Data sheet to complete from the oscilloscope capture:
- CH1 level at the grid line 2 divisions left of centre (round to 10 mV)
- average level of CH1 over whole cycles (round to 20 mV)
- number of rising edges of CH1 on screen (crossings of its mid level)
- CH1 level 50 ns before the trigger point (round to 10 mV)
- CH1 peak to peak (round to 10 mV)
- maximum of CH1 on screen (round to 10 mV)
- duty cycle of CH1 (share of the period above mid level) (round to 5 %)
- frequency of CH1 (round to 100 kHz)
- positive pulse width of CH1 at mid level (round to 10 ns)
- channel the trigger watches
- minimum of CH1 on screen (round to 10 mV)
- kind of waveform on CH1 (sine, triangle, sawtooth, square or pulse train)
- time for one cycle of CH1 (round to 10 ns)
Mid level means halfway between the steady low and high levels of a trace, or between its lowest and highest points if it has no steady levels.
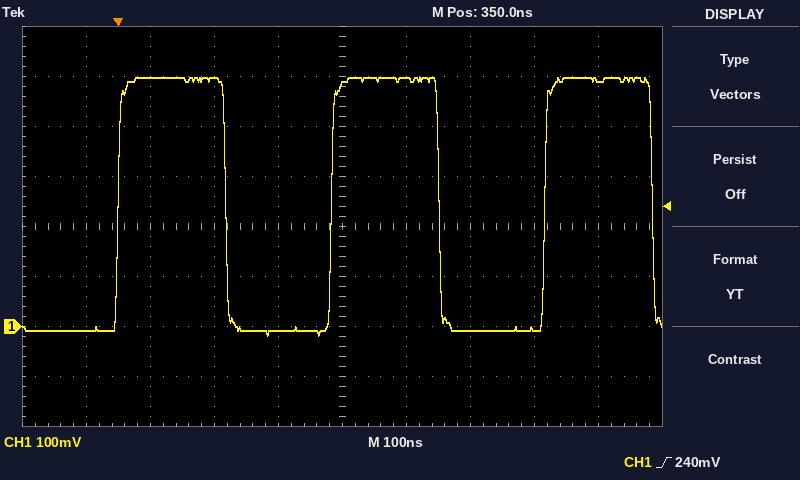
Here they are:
500 mV
240 mV
3
-10 mV
520 mV
500 mV
50 %
3.0 MHz
170 ns
CH1
-20 mV
square
330 ns
